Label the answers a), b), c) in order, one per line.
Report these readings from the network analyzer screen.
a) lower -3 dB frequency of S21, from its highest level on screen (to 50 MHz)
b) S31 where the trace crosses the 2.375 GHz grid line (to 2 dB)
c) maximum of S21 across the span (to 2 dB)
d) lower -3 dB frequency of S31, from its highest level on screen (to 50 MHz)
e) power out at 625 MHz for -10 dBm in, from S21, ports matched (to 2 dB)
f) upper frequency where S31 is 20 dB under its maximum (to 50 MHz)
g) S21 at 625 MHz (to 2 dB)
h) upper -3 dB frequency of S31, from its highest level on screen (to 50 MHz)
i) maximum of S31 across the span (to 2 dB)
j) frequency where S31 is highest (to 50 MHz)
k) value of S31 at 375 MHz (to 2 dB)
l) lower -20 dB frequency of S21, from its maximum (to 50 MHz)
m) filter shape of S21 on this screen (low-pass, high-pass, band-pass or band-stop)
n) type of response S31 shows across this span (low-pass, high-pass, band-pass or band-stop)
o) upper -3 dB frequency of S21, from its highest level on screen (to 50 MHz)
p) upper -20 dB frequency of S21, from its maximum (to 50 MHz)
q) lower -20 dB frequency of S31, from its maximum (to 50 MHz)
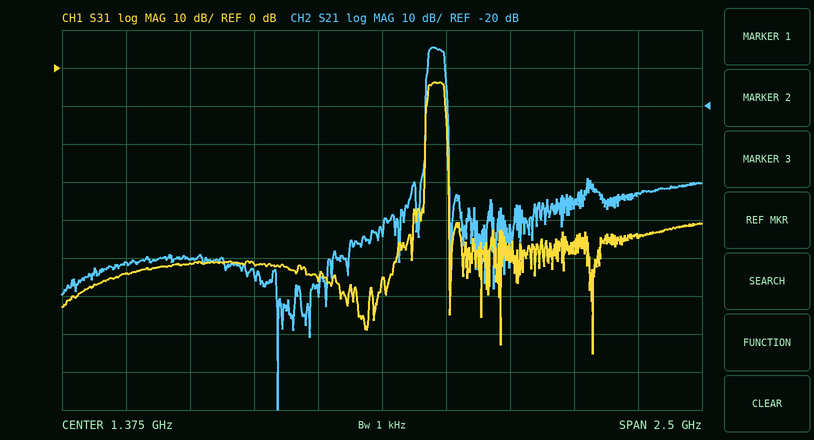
a) 1.55 GHz
b) -44 dB
c) -4 dB
d) 1.55 GHz
e) -70 dBm
f) 1.65 GHz
g) -60 dB
h) 1.60 GHz
i) -4 dB
j) 1.60 GHz
k) -54 dB
l) 1.55 GHz
m) band-pass
n) band-pass
o) 1.60 GHz
p) 1.65 GHz
q) 1.55 GHz
